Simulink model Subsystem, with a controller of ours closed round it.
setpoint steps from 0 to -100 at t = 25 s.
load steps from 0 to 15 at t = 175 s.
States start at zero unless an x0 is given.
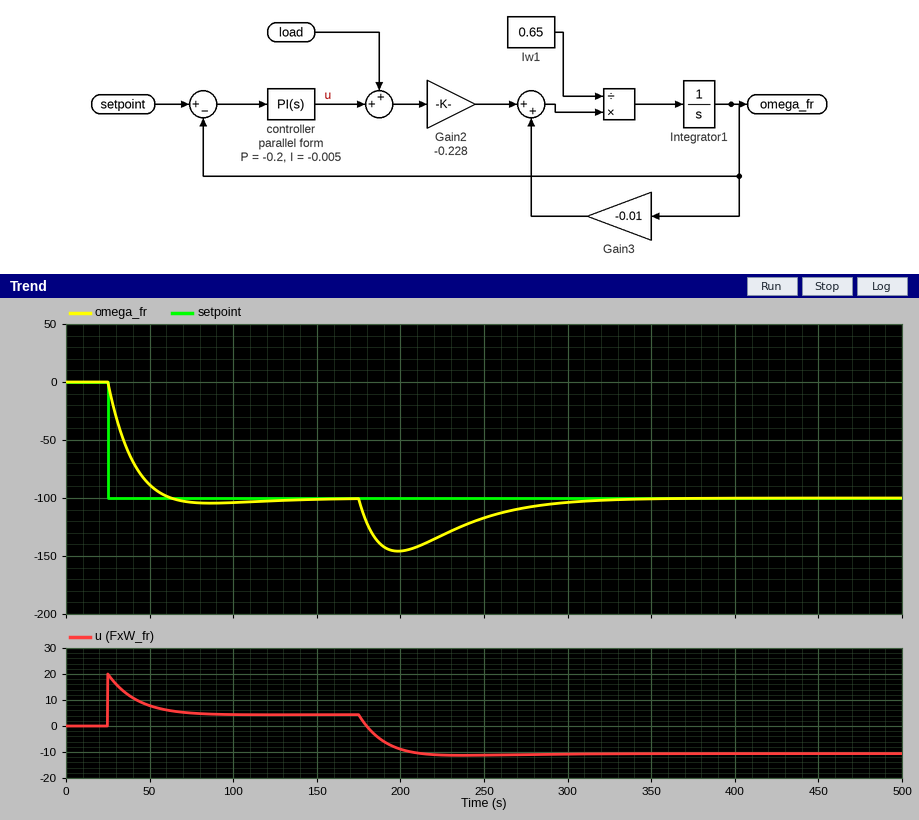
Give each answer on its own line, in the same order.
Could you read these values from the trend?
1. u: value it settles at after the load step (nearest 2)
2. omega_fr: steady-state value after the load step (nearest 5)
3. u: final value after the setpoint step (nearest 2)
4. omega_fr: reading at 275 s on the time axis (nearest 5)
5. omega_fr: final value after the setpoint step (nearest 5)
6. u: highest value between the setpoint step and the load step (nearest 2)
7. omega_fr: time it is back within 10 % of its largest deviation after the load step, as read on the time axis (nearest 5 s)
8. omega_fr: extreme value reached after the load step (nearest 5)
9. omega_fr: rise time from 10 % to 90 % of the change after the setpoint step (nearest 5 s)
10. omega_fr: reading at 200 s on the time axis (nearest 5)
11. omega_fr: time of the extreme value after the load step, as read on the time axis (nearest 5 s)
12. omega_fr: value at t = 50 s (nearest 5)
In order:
-10
-100
4
-110
-100
20
295 s
-145
25 s
-145
200 s
-90
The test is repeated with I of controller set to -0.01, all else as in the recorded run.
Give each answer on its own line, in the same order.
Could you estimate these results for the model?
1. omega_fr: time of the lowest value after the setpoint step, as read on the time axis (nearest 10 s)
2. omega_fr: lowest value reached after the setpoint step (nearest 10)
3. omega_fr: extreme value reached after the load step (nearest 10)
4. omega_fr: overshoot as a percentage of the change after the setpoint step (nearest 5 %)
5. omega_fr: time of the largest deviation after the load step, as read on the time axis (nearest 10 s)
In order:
70 s
-110
-140
15 %
190 s
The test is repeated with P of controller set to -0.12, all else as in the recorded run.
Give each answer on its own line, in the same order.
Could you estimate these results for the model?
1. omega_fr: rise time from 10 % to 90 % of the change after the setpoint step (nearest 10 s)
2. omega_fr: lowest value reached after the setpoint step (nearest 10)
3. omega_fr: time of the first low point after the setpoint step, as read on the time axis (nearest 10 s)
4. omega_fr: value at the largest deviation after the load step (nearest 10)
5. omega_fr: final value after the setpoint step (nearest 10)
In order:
30 s
-110
90 s
-160
-100
